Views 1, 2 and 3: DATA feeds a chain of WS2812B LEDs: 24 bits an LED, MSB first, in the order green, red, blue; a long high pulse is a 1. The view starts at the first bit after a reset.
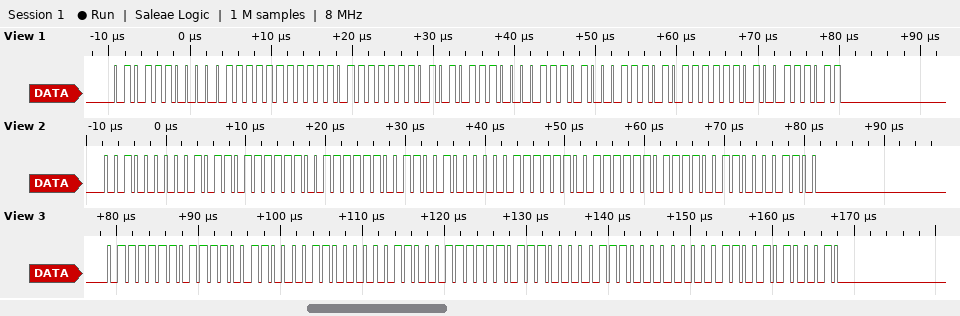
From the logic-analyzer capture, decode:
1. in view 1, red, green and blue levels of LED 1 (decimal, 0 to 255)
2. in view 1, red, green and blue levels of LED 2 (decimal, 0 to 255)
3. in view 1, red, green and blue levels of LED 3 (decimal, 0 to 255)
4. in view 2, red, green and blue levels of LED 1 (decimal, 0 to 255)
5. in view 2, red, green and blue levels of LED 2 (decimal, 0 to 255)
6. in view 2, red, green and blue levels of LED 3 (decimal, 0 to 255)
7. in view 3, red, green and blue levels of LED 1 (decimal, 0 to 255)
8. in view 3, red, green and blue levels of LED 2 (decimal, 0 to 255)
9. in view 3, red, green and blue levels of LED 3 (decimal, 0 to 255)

31, 92, 253
92, 253, 58
253, 58, 59
91, 32, 243
32, 243, 126
243, 126, 12
243, 126, 12
126, 12, 224
12, 224, 162
